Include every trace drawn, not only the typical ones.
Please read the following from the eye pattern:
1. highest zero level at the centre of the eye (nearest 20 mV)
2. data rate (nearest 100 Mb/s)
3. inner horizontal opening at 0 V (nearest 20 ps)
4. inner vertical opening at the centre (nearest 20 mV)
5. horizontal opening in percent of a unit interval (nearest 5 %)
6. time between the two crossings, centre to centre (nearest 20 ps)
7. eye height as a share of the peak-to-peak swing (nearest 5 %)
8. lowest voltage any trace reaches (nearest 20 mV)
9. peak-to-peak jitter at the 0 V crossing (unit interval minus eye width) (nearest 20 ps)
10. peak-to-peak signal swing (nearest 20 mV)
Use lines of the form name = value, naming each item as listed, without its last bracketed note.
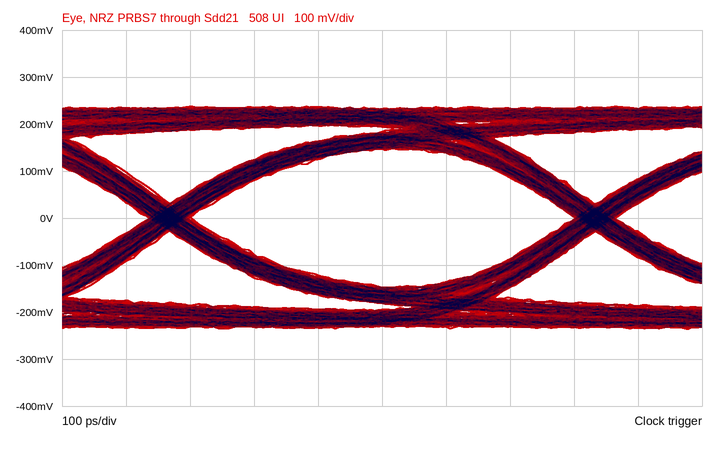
highest zero level at the centre of the eye = -140 mV
data rate = 1.5 Gb/s
inner horizontal opening at 0 V = 600 ps
inner vertical opening at the centre = 300 mV
horizontal opening in percent of a unit interval = 90 %
time between the two crossings, centre to centre = 660 ps
eye height as a share of the peak-to-peak swing = 60 %
lowest voltage any trace reaches = -240 mV
peak-to-peak jitter at the 0 V crossing (unit interval minus eye width) = 60 ps
peak-to-peak signal swing = 480 mV
